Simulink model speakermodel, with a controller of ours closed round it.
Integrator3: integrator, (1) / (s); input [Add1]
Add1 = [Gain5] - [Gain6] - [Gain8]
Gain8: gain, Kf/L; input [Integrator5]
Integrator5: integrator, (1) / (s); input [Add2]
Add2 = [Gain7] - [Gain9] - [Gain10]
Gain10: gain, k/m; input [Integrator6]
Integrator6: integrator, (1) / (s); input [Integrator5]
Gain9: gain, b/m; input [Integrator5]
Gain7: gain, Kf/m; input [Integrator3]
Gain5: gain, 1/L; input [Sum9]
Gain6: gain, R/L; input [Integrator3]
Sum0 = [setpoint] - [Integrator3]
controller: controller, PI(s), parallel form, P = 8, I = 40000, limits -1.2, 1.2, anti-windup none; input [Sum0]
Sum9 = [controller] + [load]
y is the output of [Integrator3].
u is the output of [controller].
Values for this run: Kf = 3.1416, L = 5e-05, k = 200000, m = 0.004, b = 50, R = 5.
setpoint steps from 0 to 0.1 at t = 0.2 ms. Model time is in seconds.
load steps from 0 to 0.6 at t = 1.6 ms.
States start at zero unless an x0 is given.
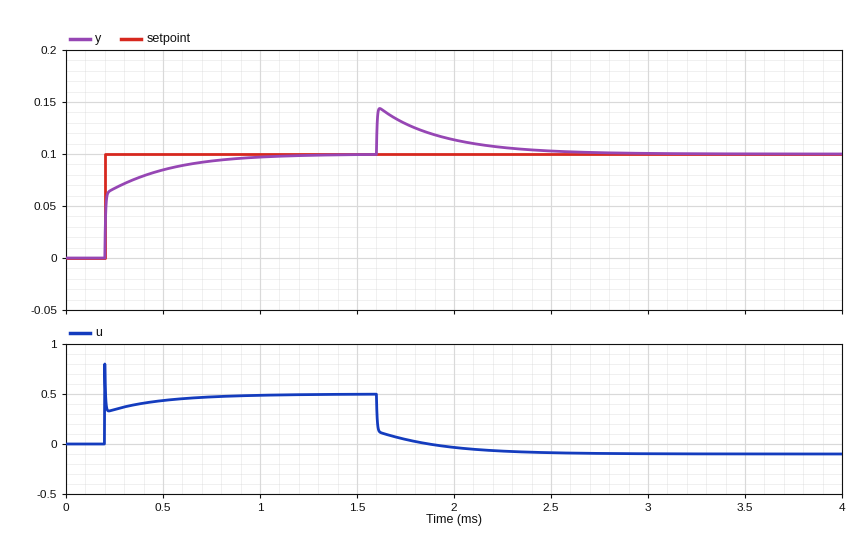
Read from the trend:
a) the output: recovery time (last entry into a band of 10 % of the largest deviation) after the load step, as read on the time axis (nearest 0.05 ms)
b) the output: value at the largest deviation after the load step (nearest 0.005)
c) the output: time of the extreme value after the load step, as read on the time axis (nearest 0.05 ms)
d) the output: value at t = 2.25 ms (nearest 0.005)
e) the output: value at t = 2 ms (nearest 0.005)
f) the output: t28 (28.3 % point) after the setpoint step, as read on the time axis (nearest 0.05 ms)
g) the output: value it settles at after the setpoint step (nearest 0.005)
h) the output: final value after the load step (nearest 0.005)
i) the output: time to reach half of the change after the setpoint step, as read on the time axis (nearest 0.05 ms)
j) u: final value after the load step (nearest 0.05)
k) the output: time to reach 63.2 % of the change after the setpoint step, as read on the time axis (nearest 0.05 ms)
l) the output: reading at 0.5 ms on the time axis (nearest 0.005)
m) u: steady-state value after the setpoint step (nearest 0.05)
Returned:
2.35 ms
0.145
1.60 ms
0.105
0.115
0.20 ms
0.100
0.100
0.20 ms
-0.10
0.20 ms
0.085
0.50
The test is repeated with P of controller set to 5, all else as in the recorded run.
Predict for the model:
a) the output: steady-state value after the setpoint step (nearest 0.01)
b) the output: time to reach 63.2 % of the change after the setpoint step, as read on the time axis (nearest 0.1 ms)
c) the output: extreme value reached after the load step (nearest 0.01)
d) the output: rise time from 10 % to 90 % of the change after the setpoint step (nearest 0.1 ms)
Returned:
0.10
0.3 ms
0.16
0.4 ms
